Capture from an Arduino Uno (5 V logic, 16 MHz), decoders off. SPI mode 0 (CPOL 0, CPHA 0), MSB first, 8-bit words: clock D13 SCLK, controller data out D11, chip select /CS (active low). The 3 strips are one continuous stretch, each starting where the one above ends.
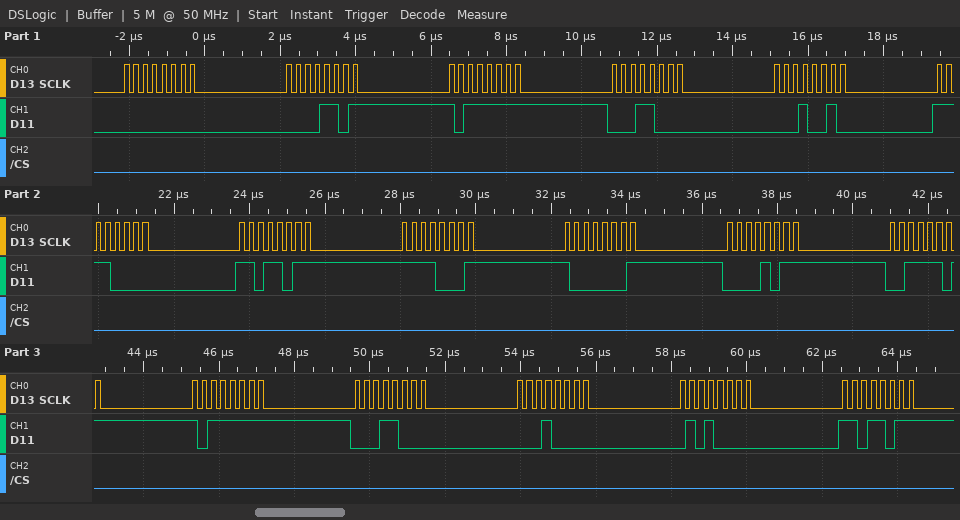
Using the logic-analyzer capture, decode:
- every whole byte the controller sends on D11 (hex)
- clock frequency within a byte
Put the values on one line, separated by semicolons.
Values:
00 0D BF 18 12 F0 DB F1 81 0B 3D BF 18 10 50 DB; 4 MHz
